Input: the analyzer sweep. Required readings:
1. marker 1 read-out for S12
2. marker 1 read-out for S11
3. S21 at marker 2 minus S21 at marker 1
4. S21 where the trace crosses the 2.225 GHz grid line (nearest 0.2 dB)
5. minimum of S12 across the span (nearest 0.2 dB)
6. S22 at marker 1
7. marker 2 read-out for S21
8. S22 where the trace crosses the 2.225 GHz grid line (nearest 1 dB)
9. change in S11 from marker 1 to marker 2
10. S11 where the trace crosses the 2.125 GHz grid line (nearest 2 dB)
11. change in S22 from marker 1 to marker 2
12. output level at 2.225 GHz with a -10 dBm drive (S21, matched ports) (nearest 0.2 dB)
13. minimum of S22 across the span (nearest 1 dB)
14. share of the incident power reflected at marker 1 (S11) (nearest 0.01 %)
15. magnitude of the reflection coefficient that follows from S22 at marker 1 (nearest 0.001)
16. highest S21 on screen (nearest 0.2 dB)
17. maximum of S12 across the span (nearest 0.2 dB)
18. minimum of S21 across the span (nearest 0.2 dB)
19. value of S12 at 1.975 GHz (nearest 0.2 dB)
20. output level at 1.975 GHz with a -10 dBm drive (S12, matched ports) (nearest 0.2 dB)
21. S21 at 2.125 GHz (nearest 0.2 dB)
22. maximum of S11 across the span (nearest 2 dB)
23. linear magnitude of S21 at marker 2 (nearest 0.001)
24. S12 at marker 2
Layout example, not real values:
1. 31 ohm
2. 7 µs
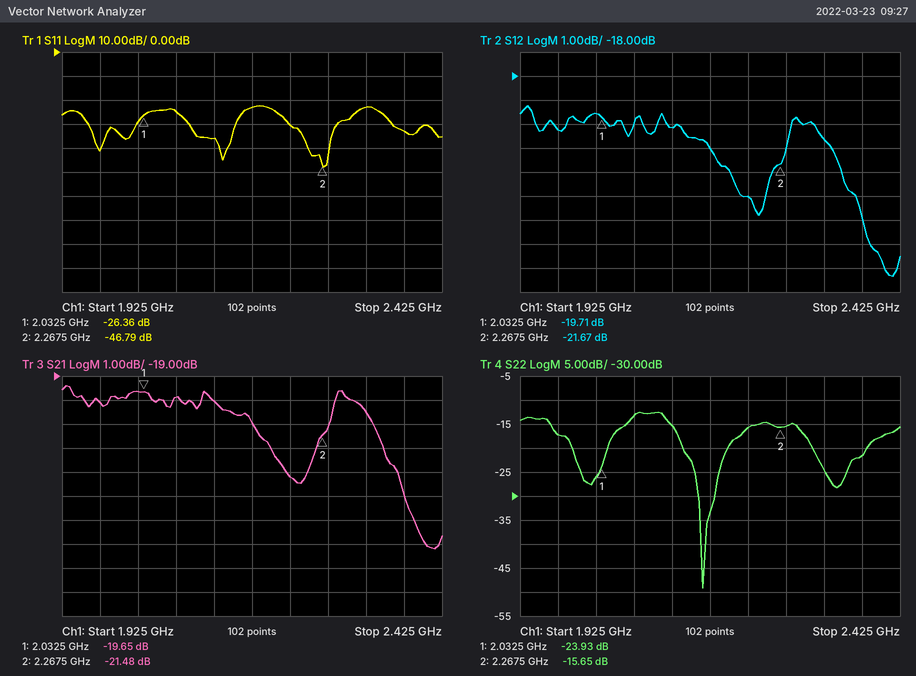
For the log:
1. -19.71 dB
2. -26.36 dB
3. -1.83 dB
4. -23.2 dB
5. -26.4 dB
6. -23.93 dB
7. -21.48 dB
8. -16 dB
9. -20.43 dB
10. -36 dB
11. 8.28 dB
12. -33.2 dBm
13. -49 dB
14. 0.23 %
15. 0.064
16. -19.4 dB
17. -19.2 dB
18. -26.2 dB
19. -20.2 dB
20. -30.2 dBm
21. -20.0 dB
22. -22 dB
23. 0.084
24. -21.67 dB
